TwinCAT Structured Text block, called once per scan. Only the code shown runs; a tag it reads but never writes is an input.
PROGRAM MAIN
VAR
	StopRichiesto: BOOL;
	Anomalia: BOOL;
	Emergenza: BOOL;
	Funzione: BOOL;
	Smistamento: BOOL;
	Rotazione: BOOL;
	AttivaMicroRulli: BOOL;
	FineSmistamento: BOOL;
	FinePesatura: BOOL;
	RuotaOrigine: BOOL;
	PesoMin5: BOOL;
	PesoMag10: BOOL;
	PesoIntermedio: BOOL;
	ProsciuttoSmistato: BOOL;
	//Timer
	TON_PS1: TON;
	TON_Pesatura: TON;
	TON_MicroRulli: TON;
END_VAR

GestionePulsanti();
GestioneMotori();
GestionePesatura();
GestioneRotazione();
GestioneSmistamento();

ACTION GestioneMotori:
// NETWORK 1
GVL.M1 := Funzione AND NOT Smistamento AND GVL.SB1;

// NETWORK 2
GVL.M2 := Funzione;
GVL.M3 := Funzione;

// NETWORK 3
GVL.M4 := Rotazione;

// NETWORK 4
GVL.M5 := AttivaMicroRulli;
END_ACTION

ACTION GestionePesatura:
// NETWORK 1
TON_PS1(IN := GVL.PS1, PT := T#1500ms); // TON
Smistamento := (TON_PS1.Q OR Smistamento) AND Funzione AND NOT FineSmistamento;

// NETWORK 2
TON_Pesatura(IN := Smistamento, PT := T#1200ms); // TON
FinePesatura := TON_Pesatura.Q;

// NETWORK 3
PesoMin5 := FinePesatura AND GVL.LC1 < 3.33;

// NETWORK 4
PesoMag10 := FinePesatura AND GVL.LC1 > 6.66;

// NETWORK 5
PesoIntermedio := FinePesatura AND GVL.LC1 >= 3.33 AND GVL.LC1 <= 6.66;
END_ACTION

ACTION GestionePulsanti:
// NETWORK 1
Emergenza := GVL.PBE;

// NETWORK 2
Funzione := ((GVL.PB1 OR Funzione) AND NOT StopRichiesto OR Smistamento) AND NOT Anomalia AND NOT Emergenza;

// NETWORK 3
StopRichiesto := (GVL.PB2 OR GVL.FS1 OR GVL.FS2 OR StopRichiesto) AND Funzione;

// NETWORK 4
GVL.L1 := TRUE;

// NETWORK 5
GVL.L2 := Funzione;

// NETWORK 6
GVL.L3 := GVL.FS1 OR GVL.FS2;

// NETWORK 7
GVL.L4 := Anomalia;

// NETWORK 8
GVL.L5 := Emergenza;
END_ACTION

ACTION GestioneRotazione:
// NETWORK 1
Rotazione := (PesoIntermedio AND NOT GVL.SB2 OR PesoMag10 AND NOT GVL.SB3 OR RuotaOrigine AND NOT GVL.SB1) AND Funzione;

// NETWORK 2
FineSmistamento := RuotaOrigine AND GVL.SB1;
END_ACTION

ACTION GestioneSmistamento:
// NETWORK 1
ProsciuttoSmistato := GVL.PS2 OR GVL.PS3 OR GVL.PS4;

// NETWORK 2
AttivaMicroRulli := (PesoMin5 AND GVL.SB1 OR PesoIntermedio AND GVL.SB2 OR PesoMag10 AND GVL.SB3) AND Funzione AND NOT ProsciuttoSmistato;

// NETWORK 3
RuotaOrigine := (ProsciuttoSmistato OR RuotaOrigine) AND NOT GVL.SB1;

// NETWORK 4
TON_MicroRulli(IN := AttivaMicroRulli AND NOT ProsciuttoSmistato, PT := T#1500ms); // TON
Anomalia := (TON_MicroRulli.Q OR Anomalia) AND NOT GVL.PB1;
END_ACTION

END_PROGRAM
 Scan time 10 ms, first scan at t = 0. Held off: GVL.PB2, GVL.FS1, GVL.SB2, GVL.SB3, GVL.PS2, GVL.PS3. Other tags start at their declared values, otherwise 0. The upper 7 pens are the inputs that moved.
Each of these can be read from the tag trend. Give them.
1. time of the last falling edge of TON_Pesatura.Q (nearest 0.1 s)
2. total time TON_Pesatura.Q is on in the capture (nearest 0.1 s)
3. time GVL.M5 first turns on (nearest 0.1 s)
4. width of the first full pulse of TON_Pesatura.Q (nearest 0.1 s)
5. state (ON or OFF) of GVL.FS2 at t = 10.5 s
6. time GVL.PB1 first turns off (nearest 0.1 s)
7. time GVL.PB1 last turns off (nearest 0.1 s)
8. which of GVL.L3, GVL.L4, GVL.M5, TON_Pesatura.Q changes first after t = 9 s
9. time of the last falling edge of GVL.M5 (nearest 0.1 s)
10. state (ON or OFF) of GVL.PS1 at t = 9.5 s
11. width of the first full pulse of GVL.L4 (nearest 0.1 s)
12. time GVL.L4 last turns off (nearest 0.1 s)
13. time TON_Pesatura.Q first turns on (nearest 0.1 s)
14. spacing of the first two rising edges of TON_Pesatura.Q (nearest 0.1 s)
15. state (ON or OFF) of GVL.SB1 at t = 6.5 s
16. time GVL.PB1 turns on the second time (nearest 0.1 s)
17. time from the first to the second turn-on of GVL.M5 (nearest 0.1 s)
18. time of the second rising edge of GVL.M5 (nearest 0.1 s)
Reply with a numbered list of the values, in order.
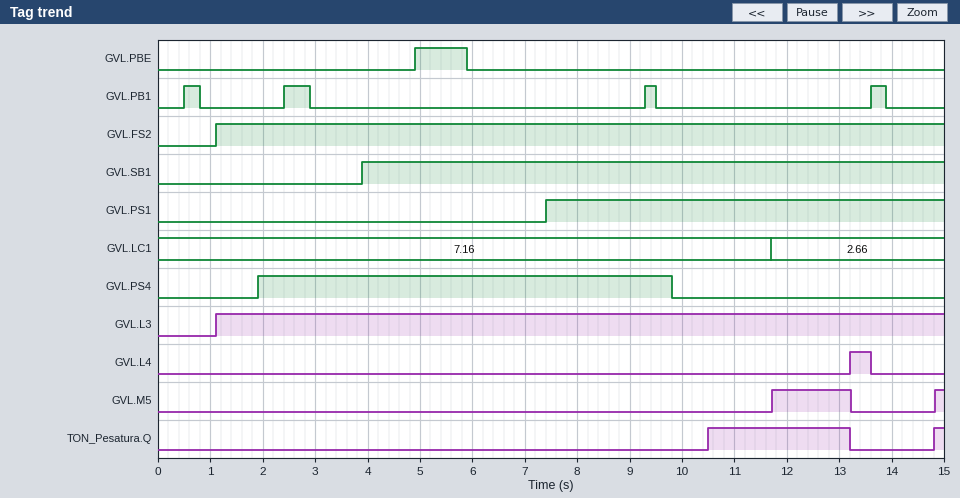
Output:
1. 13.2 s
2. 2.9 s
3. 11.7 s
4. 2.7 s
5. ON
6. 0.8 s
7. 13.9 s
8. TON_Pesatura.Q
9. 13.2 s
10. ON
11. 0.4 s
12. 13.6 s
13. 10.5 s
14. 4.3 s
15. ON
16. 2.4 s
17. 3.1 s
18. 14.8 s
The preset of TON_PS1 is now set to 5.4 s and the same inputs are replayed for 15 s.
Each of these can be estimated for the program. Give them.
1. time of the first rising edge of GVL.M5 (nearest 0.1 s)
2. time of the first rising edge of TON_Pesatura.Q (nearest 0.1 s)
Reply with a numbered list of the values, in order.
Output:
1. 14.8 s
2. 14.8 s
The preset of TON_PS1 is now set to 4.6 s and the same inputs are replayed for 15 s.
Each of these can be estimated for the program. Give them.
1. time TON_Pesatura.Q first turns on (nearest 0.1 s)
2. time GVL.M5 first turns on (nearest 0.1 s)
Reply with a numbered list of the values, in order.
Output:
1. 14.8 s
2. 14.8 s
